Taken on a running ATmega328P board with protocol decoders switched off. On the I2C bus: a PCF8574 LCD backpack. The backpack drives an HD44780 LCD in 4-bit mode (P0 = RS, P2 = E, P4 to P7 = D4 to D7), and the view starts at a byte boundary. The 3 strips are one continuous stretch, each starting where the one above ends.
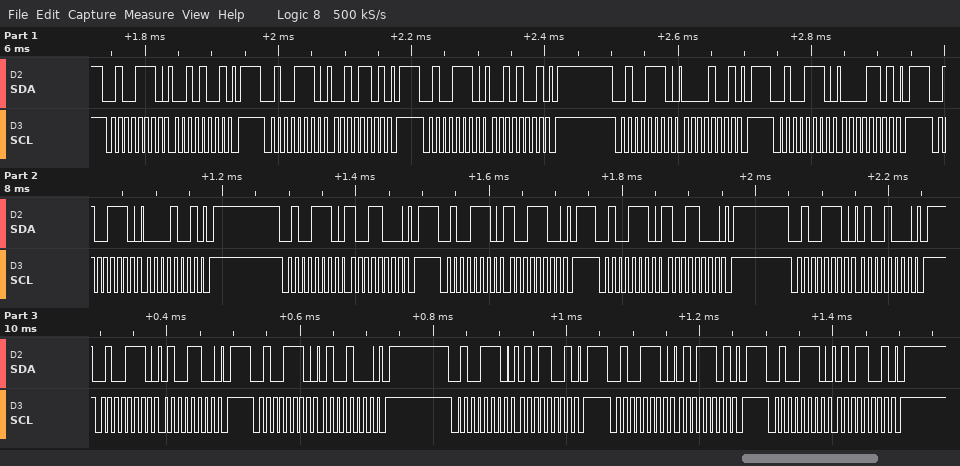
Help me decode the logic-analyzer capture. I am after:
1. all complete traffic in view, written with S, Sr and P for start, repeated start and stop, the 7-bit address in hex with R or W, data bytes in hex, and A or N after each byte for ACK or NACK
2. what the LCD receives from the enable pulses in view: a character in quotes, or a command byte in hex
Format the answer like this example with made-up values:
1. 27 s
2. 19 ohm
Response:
1. S 27W A 29 A P S 27W A 2D A P S 27W A 29 A P S 27W A 09 A P S 27W A 0D A P S 27W A 09 A P S 27W A 98 A P S 27W A 9C A P S 27W A 98 A P S 27W A 48 A P S 27W A 4C A P S 27W A 48 A P S 27W A 59 A P S 27W A 5D A P S 27W A 59 A P
2. ' ' 0x94
